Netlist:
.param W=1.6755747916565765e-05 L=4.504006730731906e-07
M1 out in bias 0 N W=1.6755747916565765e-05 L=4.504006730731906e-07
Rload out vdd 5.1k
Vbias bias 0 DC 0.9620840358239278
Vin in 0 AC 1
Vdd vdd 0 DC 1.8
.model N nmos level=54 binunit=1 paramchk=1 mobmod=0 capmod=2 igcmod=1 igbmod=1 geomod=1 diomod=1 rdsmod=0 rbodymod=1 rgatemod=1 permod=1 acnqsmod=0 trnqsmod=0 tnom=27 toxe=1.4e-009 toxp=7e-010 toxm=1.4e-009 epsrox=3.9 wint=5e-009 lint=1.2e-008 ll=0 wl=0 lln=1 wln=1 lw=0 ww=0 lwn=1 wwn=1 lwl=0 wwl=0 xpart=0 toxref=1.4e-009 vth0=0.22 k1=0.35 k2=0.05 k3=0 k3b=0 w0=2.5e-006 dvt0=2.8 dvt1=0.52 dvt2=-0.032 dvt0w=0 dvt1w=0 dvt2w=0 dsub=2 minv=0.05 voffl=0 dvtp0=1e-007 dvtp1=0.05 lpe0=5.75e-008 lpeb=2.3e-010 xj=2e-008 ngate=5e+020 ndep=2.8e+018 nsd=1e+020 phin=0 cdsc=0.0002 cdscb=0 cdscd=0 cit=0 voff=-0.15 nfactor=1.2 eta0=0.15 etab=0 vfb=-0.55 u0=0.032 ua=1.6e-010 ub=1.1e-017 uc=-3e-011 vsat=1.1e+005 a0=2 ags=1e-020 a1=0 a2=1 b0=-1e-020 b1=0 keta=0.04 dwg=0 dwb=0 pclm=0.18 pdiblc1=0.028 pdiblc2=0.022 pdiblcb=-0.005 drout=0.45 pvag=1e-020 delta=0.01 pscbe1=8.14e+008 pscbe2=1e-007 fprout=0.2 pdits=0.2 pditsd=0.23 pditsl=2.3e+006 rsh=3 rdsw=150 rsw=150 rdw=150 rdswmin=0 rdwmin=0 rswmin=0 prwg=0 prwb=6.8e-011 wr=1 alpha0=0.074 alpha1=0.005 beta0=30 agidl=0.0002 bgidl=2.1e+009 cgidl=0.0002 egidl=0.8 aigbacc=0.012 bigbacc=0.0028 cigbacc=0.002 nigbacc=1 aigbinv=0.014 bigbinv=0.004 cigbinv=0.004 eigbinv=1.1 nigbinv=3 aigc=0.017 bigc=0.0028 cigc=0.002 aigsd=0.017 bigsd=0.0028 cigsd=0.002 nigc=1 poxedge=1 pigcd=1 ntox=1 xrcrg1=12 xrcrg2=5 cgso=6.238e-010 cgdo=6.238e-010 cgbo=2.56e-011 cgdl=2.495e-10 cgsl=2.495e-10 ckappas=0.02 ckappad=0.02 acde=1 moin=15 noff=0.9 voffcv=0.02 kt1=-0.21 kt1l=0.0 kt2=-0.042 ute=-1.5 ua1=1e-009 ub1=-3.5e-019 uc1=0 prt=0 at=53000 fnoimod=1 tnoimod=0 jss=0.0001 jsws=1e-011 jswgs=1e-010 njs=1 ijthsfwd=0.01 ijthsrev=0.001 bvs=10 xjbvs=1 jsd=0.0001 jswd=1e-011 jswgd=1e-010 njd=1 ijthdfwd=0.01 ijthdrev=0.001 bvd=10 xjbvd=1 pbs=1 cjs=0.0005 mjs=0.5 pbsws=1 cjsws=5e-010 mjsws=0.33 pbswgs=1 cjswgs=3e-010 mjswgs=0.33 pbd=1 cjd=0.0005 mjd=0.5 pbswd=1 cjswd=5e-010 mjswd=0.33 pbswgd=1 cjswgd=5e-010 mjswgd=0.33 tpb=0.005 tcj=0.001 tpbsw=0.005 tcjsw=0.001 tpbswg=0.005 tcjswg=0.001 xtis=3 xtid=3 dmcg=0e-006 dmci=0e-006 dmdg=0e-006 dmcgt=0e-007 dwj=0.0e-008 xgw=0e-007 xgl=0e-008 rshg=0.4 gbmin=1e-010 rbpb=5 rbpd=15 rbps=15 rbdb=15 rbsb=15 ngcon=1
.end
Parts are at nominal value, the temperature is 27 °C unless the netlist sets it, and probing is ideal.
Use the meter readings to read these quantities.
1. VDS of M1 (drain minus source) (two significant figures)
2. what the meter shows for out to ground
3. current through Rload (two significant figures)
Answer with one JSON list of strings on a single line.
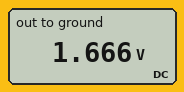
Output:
["700 mV", "1.666 V", "26 µA"]
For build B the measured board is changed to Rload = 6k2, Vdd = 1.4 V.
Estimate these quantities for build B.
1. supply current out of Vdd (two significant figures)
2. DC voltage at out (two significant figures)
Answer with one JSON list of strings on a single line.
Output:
["320 nA", "1.4 V"]
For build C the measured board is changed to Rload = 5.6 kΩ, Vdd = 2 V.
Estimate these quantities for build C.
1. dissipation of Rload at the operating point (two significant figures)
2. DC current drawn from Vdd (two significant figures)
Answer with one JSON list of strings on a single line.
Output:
["14 µW", "50 µA"]
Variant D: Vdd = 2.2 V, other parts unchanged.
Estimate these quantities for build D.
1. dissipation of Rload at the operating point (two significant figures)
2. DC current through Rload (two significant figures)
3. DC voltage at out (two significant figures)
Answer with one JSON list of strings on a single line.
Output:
["37 µW", "85 µA", "1.8 V"]
